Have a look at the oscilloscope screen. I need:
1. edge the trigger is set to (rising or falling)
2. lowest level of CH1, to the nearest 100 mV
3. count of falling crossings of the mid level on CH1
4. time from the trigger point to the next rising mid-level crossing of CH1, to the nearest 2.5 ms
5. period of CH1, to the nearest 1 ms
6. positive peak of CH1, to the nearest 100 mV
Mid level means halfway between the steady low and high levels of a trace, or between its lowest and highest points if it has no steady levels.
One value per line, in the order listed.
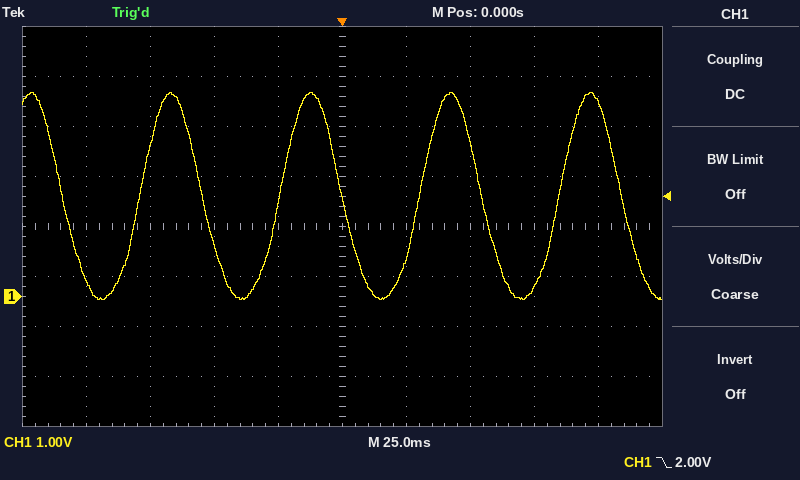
falling
-100 mV
5
30.0 ms
55 ms
4.1 V
